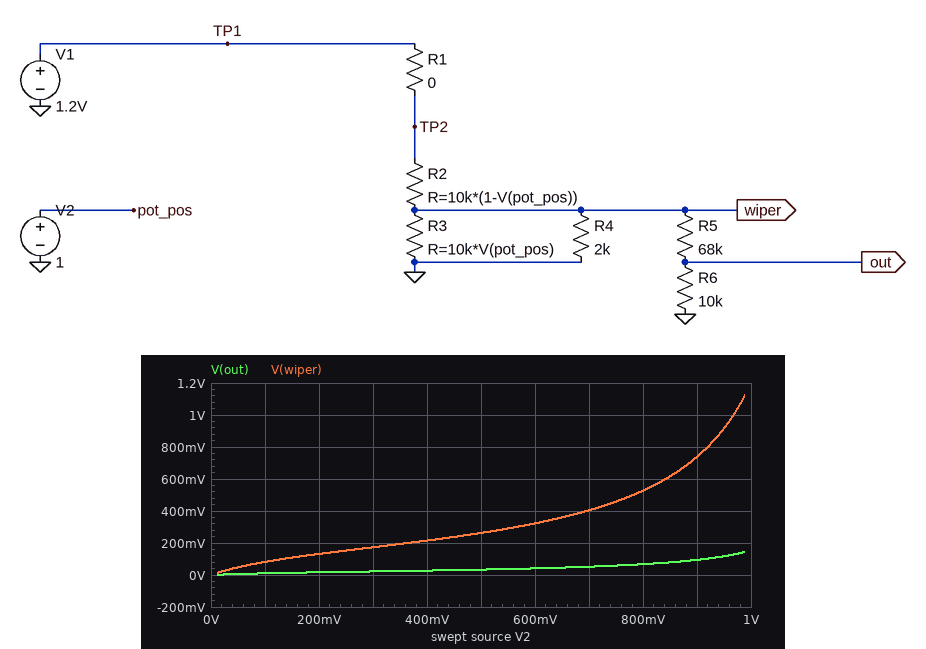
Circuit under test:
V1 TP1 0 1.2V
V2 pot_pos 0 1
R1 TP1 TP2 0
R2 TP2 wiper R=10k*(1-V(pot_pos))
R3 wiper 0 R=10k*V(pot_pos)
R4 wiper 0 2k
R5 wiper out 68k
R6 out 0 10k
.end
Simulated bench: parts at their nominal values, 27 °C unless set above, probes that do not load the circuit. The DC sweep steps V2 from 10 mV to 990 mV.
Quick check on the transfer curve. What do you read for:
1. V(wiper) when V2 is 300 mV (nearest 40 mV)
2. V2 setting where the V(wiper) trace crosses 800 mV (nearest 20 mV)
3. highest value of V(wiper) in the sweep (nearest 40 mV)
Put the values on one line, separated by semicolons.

160 mV; 920 mV; 1.12 V
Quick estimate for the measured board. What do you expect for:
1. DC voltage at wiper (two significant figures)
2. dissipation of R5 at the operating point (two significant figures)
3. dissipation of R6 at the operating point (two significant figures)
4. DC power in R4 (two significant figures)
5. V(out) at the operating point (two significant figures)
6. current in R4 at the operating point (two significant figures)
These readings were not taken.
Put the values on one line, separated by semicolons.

1.2 V; 16 µW; 2.4 µW; 720 µW; 150 mV; 600 µA
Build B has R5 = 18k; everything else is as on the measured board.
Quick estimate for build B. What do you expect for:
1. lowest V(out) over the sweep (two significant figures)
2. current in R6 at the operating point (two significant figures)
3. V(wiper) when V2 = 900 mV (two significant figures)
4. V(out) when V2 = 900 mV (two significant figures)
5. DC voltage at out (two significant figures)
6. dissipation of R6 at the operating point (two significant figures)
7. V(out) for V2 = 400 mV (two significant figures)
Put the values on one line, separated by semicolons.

4.1 mV; 43 µA; 730 mV; 260 mV; 430 mV; 18 µW; 75 mV
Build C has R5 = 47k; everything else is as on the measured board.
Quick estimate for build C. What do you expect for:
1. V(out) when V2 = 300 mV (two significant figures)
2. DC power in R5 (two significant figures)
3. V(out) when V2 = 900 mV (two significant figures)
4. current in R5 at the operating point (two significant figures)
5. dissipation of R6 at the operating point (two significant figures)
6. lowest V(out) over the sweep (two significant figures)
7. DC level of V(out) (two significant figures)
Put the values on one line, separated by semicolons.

30 mV; 21 µW; 130 mV; 21 µA; 4.4 µW; 2.0 mV; 210 mV
